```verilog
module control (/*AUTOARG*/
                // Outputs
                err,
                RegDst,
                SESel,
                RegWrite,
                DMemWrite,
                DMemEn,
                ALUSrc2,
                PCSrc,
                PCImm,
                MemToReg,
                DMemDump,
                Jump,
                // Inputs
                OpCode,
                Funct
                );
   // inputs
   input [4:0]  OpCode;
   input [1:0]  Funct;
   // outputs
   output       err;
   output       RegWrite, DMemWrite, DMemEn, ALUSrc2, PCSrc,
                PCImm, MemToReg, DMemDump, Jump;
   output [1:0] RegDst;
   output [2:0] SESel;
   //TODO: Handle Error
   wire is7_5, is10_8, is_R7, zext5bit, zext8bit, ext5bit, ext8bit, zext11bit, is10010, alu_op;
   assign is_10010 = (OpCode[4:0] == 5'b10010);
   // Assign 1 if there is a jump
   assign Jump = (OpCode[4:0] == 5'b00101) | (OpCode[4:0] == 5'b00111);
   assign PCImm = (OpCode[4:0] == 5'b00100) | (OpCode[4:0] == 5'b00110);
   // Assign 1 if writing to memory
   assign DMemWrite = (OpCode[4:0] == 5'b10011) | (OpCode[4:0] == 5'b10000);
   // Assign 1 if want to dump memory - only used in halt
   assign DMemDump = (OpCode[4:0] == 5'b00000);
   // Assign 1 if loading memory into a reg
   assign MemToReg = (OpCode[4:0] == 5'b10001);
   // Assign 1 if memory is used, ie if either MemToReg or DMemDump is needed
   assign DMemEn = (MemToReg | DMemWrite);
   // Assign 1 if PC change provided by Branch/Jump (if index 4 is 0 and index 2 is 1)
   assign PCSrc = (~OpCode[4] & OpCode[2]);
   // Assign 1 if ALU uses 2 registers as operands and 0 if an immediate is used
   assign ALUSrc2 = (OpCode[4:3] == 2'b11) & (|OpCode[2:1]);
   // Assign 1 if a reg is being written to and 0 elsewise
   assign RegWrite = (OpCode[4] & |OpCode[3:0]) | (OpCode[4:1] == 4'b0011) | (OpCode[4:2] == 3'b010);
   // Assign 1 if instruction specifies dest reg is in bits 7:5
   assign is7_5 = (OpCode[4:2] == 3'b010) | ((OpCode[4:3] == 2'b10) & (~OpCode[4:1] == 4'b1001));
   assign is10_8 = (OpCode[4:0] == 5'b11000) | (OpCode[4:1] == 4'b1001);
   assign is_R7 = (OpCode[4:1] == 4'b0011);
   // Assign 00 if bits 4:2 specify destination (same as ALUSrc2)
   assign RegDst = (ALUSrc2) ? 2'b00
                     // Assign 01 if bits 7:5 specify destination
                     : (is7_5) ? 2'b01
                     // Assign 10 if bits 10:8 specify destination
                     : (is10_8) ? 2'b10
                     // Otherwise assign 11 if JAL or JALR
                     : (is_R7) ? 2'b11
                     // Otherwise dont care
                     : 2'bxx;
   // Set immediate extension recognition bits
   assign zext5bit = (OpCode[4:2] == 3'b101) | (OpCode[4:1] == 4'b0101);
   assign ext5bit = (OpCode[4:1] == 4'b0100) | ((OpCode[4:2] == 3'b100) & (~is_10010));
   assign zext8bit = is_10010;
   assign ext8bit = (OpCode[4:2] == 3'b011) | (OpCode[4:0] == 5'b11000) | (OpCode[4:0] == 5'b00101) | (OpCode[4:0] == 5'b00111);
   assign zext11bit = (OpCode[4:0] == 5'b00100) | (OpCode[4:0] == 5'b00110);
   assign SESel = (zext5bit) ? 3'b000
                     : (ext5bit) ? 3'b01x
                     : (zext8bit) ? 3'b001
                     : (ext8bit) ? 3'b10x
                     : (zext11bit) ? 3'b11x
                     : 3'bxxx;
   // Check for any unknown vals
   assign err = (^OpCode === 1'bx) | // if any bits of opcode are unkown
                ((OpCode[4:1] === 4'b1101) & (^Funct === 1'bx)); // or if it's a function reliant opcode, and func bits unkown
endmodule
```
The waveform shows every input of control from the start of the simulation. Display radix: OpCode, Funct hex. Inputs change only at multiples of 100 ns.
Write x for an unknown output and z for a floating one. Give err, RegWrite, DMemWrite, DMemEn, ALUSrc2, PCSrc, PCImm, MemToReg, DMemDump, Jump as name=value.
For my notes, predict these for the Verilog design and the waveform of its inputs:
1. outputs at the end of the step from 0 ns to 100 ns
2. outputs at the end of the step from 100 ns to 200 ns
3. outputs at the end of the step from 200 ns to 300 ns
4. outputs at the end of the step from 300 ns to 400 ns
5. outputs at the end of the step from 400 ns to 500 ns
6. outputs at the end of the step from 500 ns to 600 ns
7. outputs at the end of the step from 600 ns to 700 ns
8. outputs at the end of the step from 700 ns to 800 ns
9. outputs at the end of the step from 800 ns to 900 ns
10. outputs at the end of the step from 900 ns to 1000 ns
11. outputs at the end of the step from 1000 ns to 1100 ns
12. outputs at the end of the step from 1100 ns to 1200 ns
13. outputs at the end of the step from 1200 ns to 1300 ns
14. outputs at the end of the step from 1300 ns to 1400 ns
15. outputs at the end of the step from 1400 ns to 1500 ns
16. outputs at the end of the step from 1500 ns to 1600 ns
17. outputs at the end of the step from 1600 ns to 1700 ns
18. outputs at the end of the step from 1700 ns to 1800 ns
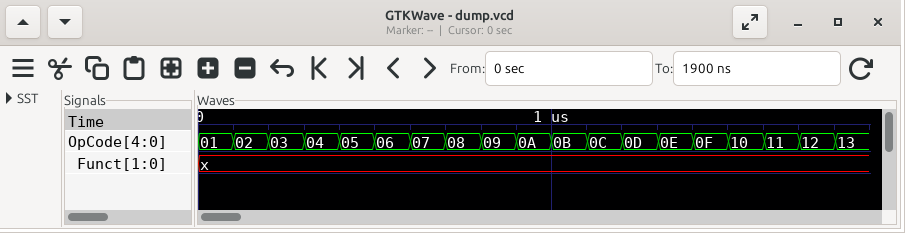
err=0, RegWrite=0, DMemWrite=0, DMemEn=0, ALUSrc2=0, PCSrc=0, PCImm=0, MemToReg=0, DMemDump=0, Jump=0
err=0, RegWrite=0, DMemWrite=0, DMemEn=0, ALUSrc2=0, PCSrc=0, PCImm=0, MemToReg=0, DMemDump=0, Jump=0
err=0, RegWrite=0, DMemWrite=0, DMemEn=0, ALUSrc2=0, PCSrc=0, PCImm=0, MemToReg=0, DMemDump=0, Jump=0
err=0, RegWrite=0, DMemWrite=0, DMemEn=0, ALUSrc2=0, PCSrc=1, PCImm=1, MemToReg=0, DMemDump=0, Jump=0
err=0, RegWrite=0, DMemWrite=0, DMemEn=0, ALUSrc2=0, PCSrc=1, PCImm=0, MemToReg=0, DMemDump=0, Jump=1
err=0, RegWrite=1, DMemWrite=0, DMemEn=0, ALUSrc2=0, PCSrc=1, PCImm=1, MemToReg=0, DMemDump=0, Jump=0
err=0, RegWrite=1, DMemWrite=0, DMemEn=0, ALUSrc2=0, PCSrc=1, PCImm=0, MemToReg=0, DMemDump=0, Jump=1
err=0, RegWrite=1, DMemWrite=0, DMemEn=0, ALUSrc2=0, PCSrc=0, PCImm=0, MemToReg=0, DMemDump=0, Jump=0
err=0, RegWrite=1, DMemWrite=0, DMemEn=0, ALUSrc2=0, PCSrc=0, PCImm=0, MemToReg=0, DMemDump=0, Jump=0
err=0, RegWrite=1, DMemWrite=0, DMemEn=0, ALUSrc2=0, PCSrc=0, PCImm=0, MemToReg=0, DMemDump=0, Jump=0
err=0, RegWrite=1, DMemWrite=0, DMemEn=0, ALUSrc2=0, PCSrc=0, PCImm=0, MemToReg=0, DMemDump=0, Jump=0
err=0, RegWrite=0, DMemWrite=0, DMemEn=0, ALUSrc2=0, PCSrc=1, PCImm=0, MemToReg=0, DMemDump=0, Jump=0
err=0, RegWrite=0, DMemWrite=0, DMemEn=0, ALUSrc2=0, PCSrc=1, PCImm=0, MemToReg=0, DMemDump=0, Jump=0
err=0, RegWrite=0, DMemWrite=0, DMemEn=0, ALUSrc2=0, PCSrc=1, PCImm=0, MemToReg=0, DMemDump=0, Jump=0
err=0, RegWrite=0, DMemWrite=0, DMemEn=0, ALUSrc2=0, PCSrc=1, PCImm=0, MemToReg=0, DMemDump=0, Jump=0
err=0, RegWrite=0, DMemWrite=1, DMemEn=1, ALUSrc2=0, PCSrc=0, PCImm=0, MemToReg=0, DMemDump=0, Jump=0
err=0, RegWrite=1, DMemWrite=0, DMemEn=1, ALUSrc2=0, PCSrc=0, PCImm=0, MemToReg=1, DMemDump=0, Jump=0
err=0, RegWrite=1, DMemWrite=0, DMemEn=0, ALUSrc2=0, PCSrc=0, PCImm=0, MemToReg=0, DMemDump=0, Jump=0
